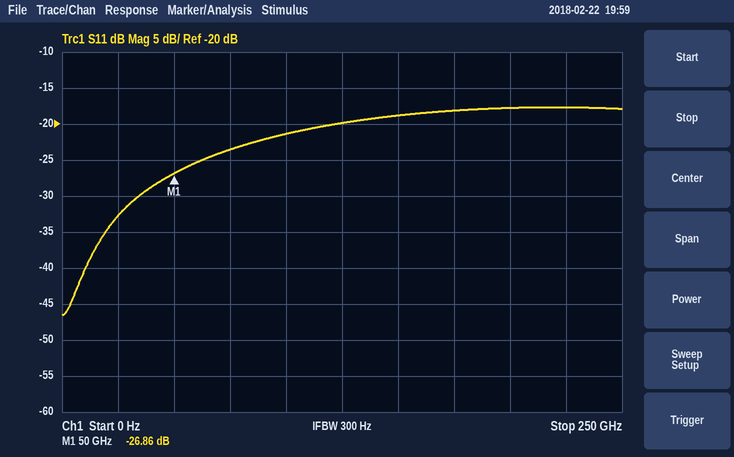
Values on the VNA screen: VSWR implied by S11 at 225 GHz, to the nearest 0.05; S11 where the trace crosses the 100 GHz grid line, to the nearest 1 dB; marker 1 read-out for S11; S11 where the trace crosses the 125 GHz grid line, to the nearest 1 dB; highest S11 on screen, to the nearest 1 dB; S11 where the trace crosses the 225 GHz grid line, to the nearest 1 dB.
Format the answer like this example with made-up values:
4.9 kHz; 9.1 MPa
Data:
1.30; -21 dB; -26.86 dB; -20 dB; -18 dB; -18 dB
